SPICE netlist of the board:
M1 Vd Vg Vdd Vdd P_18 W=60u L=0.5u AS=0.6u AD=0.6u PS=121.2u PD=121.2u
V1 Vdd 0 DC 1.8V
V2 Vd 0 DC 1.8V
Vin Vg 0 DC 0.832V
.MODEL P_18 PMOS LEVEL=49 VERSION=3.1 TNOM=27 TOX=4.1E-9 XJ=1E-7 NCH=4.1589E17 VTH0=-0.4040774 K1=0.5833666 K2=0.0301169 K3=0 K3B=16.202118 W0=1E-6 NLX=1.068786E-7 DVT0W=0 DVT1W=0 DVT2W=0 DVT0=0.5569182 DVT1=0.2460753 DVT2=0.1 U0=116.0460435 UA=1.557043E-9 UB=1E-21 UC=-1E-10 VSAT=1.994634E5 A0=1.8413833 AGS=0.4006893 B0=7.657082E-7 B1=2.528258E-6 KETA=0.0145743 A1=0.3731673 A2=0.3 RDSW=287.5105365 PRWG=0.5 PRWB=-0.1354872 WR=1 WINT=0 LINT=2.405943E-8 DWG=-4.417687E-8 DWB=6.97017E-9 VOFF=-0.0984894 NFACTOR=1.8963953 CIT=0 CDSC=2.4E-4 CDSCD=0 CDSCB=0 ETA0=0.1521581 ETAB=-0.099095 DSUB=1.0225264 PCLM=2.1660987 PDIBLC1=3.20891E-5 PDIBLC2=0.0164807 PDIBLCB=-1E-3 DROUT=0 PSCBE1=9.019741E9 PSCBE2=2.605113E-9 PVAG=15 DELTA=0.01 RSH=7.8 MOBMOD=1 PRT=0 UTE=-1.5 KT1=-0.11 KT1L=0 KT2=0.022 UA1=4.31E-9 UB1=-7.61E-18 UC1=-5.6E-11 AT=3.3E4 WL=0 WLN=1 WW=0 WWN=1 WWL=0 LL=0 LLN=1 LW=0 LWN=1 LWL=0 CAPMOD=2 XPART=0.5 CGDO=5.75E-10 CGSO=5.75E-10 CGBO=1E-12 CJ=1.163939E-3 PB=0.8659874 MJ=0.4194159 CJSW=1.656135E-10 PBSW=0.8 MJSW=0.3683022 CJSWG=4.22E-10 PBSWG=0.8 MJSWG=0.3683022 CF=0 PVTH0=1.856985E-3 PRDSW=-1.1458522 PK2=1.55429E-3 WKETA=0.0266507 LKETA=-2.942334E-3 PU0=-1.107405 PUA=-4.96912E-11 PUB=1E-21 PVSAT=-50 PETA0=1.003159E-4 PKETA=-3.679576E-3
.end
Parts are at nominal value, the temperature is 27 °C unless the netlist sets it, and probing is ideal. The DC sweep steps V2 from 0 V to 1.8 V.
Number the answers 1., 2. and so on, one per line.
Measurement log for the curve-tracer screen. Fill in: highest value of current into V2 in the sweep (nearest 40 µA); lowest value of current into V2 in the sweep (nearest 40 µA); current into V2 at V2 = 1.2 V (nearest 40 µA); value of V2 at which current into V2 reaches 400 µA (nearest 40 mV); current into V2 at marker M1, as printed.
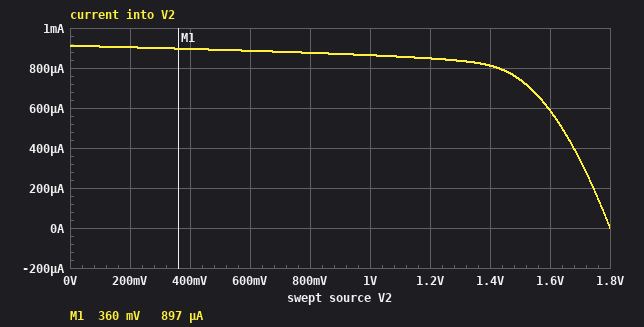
1. 920 µA
2. 0 A
3. 840 µA
4. 1.68 V
5. 897 µA
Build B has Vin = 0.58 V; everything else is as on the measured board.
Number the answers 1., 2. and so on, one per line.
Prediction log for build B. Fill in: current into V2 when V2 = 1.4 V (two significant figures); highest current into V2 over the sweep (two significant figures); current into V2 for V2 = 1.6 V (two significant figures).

1. 1.4 mA
2. 1.8 mA
3. 890 µA
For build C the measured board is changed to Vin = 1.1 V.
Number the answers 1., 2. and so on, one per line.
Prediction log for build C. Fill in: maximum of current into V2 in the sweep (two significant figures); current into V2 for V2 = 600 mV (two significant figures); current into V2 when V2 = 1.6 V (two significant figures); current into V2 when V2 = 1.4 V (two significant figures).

1. 250 µA
2. 240 µA
3. 210 µA
4. 220 µA
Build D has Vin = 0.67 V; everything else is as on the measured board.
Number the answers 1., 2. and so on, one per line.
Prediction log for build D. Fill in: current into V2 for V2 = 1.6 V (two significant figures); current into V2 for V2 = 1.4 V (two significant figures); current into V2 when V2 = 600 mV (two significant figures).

1. 790 µA
2. 1.2 mA
3. 1.4 mA
